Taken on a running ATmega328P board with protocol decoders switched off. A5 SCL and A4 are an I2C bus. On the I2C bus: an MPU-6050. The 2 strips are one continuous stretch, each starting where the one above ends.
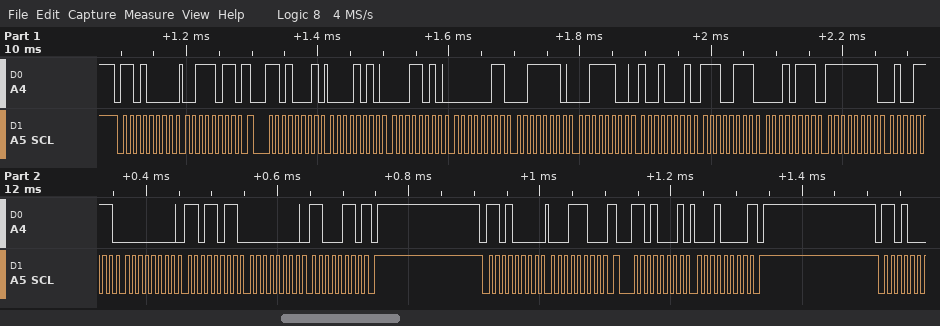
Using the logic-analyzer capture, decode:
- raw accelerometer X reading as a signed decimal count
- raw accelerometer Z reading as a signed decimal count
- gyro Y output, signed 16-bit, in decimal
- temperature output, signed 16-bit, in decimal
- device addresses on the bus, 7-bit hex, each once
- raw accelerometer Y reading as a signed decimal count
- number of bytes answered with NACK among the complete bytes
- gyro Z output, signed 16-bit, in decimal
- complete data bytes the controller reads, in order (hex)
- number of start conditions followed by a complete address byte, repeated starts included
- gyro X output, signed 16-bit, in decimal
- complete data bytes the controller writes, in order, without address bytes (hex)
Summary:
2586
15505
219
-6377
0x68
830
2
198
0A 1A 03 3E 3C 91 E7 17 FF 4F 00 DB 00 C6 10
4
-177
3B 1C
